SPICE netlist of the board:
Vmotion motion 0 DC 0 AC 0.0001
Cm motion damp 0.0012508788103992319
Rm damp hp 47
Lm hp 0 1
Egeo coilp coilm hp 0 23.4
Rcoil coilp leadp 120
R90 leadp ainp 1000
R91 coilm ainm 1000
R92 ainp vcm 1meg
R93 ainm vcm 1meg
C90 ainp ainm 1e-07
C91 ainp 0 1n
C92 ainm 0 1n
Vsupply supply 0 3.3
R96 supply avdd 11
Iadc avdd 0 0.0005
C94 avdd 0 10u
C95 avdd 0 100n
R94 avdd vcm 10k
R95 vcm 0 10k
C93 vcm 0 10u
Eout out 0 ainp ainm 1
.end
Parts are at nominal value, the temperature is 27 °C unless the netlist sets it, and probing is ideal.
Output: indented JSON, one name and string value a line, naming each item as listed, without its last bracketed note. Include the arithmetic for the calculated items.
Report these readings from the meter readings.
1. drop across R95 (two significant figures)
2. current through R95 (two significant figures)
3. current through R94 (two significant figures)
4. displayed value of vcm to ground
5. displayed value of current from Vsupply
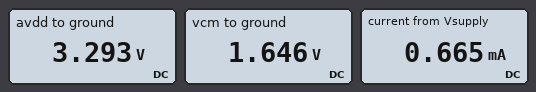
{
  "drop across R95": "1.646 V = 1.6 V",
  "current through R95": "(1.646 V) / 10 kΩ = 160 µA",
  "current through R94": "(3.293 V - 1.646 V) / 10 kΩ = 160 µA",
  "displayed value of vcm to ground": "1.646 V",
  "displayed value of current from Vsupply": "0.665 mA"
}
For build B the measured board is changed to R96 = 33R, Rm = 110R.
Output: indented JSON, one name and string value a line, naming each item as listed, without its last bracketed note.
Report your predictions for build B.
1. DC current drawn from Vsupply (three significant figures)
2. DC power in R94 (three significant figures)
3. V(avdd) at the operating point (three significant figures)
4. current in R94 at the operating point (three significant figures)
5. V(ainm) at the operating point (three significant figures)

{
  "DC current drawn from Vsupply": "664 µA",
  "DC power in R94": "269 µW",
  "V(avdd) at the operating point": "3.28 V",
  "current in R94 at the operating point": "164 µA",
  "V(ainm) at the operating point": "1.64 V"
}
